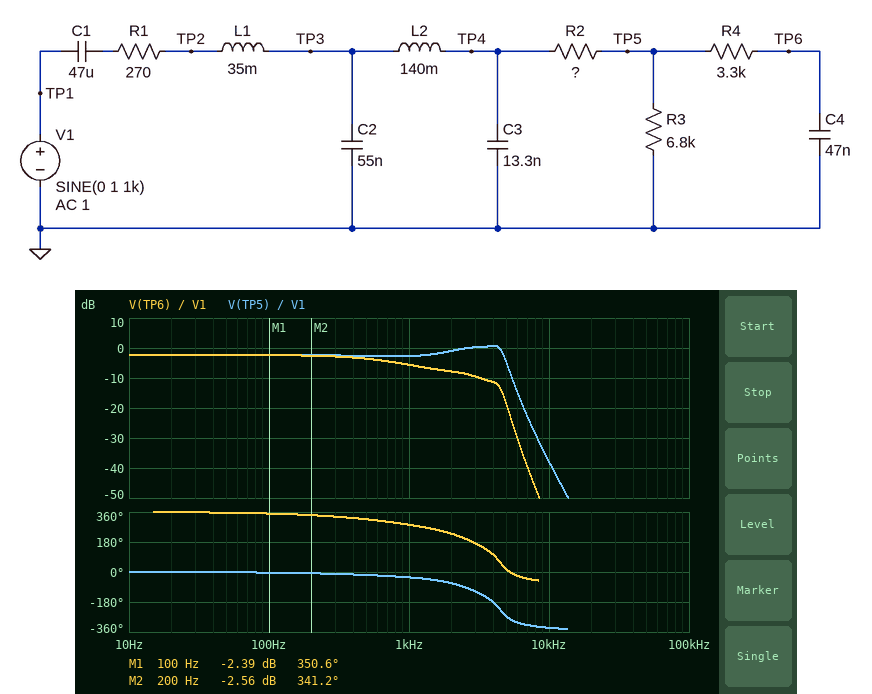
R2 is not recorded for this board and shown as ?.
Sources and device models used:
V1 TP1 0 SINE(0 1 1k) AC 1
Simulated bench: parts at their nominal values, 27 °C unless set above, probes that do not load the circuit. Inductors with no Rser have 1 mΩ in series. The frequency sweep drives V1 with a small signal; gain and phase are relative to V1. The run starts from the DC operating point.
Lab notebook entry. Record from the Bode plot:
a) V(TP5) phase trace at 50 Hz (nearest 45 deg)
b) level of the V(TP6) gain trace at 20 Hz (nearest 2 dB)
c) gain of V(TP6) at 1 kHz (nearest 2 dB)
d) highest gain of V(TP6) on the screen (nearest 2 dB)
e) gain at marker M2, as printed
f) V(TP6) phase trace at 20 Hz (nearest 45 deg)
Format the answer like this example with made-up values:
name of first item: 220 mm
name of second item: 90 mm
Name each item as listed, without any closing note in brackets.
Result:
V(TP5) phase trace at 50 Hz: 0 deg
level of the V(TP6) gain trace at 20 Hz: -2 dB
gain of V(TP6) at 1 kHz: -6 dB
highest gain of V(TP6) on the screen: -2 dB
gain at marker M2, as printed: -2.56 dB
V(TP6) phase trace at 20 Hz: 360 deg
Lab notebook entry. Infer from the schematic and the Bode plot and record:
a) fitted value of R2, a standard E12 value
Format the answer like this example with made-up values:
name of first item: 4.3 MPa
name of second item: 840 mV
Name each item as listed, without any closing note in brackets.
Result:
fitted value of R2, a standard E12 value: 1.8 kΩ
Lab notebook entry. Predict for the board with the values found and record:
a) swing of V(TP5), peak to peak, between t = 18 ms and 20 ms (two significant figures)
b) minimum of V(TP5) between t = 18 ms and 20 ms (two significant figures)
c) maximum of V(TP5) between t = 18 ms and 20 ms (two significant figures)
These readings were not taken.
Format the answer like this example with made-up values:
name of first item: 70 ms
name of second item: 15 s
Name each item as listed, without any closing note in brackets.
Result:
swing of V(TP5), peak to peak, between t = 18 ms and 20 ms: 1.5 V
minimum of V(TP5) between t = 18 ms and 20 ms: -730 mV
maximum of V(TP5) between t = 18 ms and 20 ms: 730 mV
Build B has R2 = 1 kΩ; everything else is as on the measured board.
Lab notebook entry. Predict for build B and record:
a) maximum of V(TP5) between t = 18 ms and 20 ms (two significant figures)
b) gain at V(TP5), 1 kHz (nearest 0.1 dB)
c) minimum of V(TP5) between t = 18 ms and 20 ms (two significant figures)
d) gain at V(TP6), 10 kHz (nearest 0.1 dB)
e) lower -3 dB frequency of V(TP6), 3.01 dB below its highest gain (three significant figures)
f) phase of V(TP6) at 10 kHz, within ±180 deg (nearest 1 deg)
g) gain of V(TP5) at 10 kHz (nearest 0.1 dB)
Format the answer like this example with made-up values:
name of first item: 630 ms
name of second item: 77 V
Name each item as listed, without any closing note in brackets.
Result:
maximum of V(TP5) between t = 18 ms and 20 ms: 880 mV
gain at V(TP5), 1 kHz: -1.1 dB
minimum of V(TP5) between t = 18 ms and 20 ms: -880 mV
gain at V(TP6), 10 kHz: -56.1 dB
lower -3 dB frequency of V(TP6), 3.01 dB below its highest gain: 418 mHz
phase of V(TP6) at 10 kHz, within ±180 deg: -54 deg
gain of V(TP5) at 10 kHz: -36.2 dB
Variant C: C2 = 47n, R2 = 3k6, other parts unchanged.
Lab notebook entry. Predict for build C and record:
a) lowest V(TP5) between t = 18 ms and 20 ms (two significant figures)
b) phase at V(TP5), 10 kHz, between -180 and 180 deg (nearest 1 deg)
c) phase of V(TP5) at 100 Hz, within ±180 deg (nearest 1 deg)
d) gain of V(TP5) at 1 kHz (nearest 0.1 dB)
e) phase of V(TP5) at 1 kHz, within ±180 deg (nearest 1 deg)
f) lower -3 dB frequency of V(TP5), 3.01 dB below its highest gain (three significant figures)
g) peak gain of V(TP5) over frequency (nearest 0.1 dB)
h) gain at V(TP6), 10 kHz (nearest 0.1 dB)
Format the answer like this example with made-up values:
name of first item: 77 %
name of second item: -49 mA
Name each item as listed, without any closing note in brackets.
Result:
lowest V(TP5) between t = 18 ms and 20 ms: -530 mV
phase at V(TP5), 10 kHz, between -180 and 180 deg: 19 deg
phase of V(TP5) at 100 Hz, within ±180 deg: -5 deg
gain of V(TP5) at 1 kHz: -5.5 dB
phase of V(TP5) at 1 kHz, within ±180 deg: -32 deg
lower -3 dB frequency of V(TP5), 3.01 dB below its highest gain: 1.84 kHz
peak gain of V(TP5) over frequency: -0.9 dB
gain at V(TP6), 10 kHz: -58.9 dB
